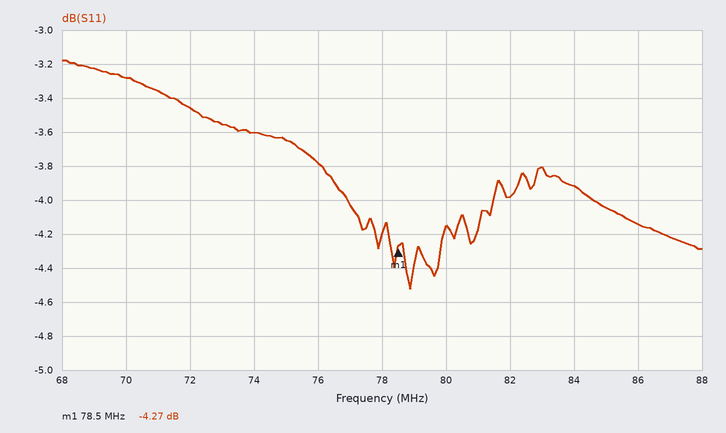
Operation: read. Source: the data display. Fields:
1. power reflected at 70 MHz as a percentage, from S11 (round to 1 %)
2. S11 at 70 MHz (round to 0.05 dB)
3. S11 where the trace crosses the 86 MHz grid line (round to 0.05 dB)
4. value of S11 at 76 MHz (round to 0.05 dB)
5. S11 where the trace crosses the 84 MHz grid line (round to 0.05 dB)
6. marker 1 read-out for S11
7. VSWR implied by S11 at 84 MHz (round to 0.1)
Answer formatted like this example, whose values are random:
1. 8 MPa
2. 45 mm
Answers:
1. 47 %
2. -3.30 dB
3. -4.15 dB
4. -3.80 dB
5. -3.90 dB
6. -4.27 dB
7. 4.5
